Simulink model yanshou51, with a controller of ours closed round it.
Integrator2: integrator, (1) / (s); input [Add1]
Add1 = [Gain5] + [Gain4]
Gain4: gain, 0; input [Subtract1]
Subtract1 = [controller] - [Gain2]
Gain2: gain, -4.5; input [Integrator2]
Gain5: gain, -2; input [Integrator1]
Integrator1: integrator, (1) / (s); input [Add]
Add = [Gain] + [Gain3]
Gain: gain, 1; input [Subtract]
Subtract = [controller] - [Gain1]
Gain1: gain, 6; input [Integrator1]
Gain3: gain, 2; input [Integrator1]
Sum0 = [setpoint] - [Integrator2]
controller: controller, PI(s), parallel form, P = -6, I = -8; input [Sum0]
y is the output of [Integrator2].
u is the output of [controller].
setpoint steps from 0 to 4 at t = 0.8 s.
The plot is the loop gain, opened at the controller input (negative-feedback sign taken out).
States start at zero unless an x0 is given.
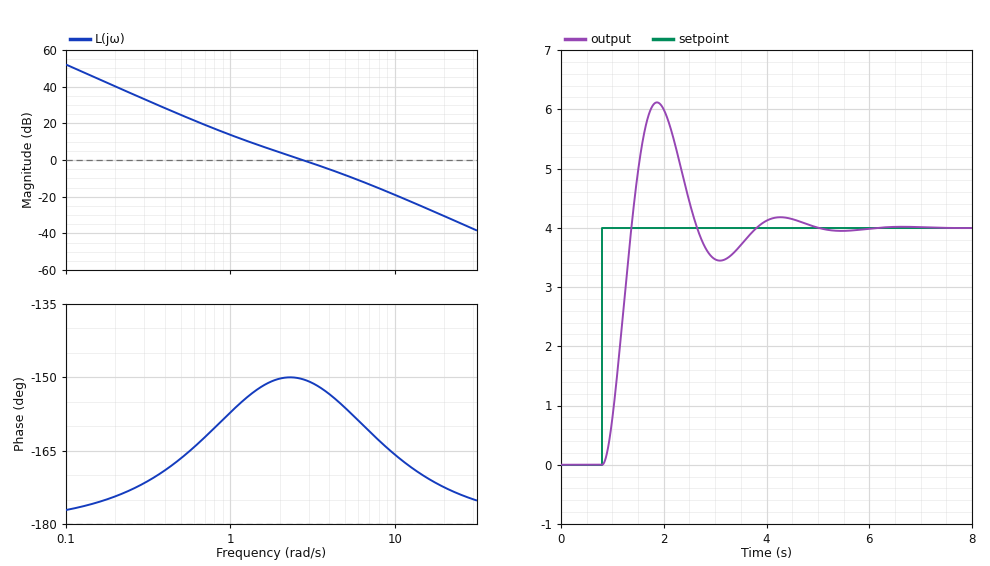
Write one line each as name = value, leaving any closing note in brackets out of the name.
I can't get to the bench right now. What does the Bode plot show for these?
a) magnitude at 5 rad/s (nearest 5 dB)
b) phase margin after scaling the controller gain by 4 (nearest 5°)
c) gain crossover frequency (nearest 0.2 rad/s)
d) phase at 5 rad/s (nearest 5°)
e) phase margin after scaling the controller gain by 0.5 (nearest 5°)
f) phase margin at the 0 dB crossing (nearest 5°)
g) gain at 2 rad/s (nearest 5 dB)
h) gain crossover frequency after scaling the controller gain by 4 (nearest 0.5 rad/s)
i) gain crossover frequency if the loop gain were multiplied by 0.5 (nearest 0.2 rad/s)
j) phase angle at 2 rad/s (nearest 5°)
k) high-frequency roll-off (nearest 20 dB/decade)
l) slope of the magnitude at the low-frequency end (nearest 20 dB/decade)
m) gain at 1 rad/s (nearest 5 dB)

magnitude at 5 rad/s = -10 dB
phase margin after scaling the controller gain by 4 = 20°
gain crossover frequency = 2.8 rad/s
phase at 5 rad/s = -155°
phase margin after scaling the controller gain by 0.5 = 30°
phase margin at the 0 dB crossing = 30°
gain at 2 rad/s = 5 dB
gain crossover frequency after scaling the controller gain by 4 = 6.5 rad/s
gain crossover frequency if the loop gain were multiplied by 0.5 = 1.8 rad/s
phase angle at 2 rad/s = -150°
high-frequency roll-off = -40 dB/decade
slope of the magnitude at the low-frequency end = -40 dB/decade
gain at 1 rad/s = 15 dB
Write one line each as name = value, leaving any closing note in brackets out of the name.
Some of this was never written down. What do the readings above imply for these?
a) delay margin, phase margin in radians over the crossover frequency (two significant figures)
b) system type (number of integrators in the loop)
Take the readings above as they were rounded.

delay margin, phase margin in radians over the crossover frequency = 0.19 s
system type = 2
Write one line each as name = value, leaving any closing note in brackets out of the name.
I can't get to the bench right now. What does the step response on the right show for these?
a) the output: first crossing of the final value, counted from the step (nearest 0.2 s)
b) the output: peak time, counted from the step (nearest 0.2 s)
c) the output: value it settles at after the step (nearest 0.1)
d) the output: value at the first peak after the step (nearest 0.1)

the output: first crossing of the final value, counted from the step = 0.6 s
the output: peak time, counted from the step = 1.0 s
the output: value it settles at after the step = 4.0
the output: value at the first peak after the step = 6.1
